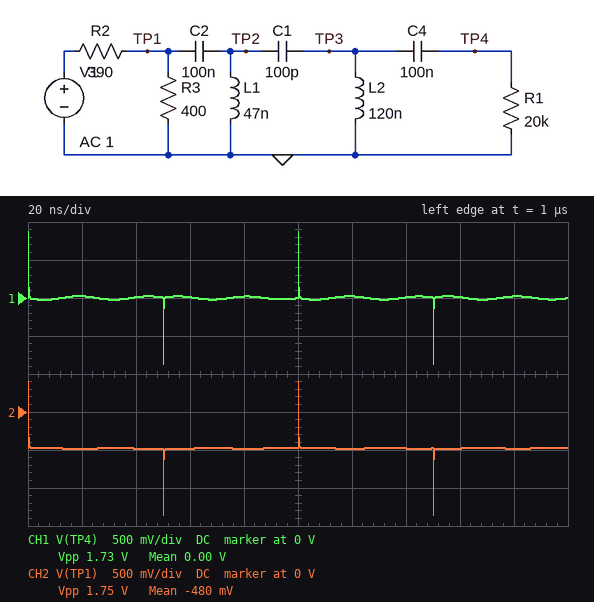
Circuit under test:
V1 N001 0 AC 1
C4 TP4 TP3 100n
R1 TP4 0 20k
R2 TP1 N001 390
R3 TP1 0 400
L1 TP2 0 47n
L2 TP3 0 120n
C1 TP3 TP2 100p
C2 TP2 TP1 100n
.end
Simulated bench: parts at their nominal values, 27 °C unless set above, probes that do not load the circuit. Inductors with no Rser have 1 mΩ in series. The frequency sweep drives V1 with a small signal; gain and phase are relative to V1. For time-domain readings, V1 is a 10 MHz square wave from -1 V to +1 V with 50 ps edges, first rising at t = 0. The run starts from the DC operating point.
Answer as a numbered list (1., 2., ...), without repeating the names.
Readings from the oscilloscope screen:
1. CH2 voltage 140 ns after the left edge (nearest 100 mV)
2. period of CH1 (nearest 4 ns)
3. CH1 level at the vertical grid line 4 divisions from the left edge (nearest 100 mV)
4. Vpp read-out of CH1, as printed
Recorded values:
1. -500 mV
2. 100 ns
3. 0 V
4. 1.73 V
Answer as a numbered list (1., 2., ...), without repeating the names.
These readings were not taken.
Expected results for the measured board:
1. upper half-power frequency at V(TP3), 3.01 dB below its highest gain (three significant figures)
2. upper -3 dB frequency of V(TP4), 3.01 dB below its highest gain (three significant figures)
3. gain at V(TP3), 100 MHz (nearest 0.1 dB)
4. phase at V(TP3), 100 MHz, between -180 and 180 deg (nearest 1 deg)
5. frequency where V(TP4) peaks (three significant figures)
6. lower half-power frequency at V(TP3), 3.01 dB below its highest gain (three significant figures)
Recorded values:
1. 39.3 MHz
2. 39.3 MHz
3. -23.9 dB
4. 84 deg
5. 39.0 MHz
6. 38.6 MHz
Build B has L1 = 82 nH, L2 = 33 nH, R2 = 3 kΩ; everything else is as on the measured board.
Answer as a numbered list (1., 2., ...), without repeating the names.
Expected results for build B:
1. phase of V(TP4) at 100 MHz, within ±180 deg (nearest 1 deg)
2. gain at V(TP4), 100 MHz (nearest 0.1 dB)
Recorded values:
1. 89 deg
2. -44.0 dB
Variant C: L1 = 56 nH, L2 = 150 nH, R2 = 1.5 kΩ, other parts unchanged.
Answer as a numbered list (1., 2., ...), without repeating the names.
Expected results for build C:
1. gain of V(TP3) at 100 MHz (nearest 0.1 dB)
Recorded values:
1. -34.2 dB
